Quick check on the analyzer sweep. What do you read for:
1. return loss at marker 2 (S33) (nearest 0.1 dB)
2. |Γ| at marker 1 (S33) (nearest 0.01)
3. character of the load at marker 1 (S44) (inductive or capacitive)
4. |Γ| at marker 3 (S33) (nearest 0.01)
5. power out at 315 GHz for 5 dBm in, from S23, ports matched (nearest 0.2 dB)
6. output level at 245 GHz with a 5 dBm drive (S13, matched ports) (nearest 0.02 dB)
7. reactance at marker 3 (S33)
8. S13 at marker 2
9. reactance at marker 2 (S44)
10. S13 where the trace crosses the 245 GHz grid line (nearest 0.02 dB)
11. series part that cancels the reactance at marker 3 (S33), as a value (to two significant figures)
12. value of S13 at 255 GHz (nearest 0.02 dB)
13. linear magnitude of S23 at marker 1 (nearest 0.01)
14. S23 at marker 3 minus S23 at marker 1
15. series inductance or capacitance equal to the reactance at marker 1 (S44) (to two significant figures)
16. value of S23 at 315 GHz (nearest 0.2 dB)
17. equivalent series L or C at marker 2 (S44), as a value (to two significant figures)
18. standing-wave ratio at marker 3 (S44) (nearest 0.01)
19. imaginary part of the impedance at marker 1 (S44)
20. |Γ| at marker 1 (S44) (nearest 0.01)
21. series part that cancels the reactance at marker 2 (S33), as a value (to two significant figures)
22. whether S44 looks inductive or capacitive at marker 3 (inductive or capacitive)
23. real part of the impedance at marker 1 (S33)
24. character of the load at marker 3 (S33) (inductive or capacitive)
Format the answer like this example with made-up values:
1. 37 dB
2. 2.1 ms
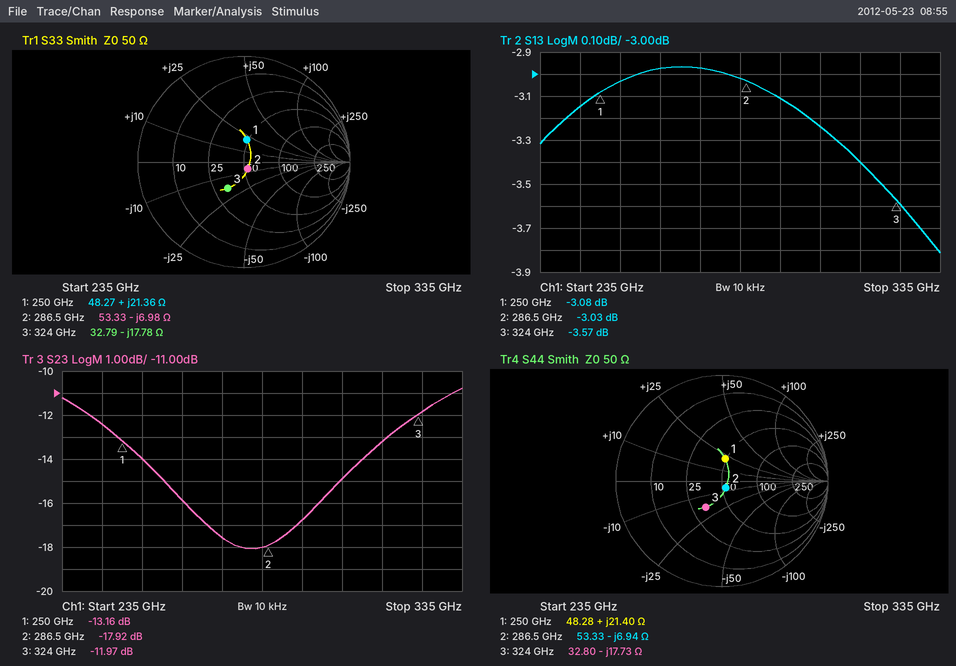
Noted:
1. 22.5 dB
2. 0.21
3. inductive
4. 0.29
5. -8.2 dBm
6. 1.86 dBm
7. -17.78 Ω
8. -3.03 dB
9. -6.94 Ω
10. -3.14 dB
11. 8.7 pH
12. -3.04 dB
13. 0.22
14. 1.19 dB
15. 14 pH
16. -13.2 dB
17. 80 fF
18. 1.82
19. +21.40 Ω
20. 0.21
21. 3.9 pH
22. capacitive
23. 48.27 Ω
24. capacitive
